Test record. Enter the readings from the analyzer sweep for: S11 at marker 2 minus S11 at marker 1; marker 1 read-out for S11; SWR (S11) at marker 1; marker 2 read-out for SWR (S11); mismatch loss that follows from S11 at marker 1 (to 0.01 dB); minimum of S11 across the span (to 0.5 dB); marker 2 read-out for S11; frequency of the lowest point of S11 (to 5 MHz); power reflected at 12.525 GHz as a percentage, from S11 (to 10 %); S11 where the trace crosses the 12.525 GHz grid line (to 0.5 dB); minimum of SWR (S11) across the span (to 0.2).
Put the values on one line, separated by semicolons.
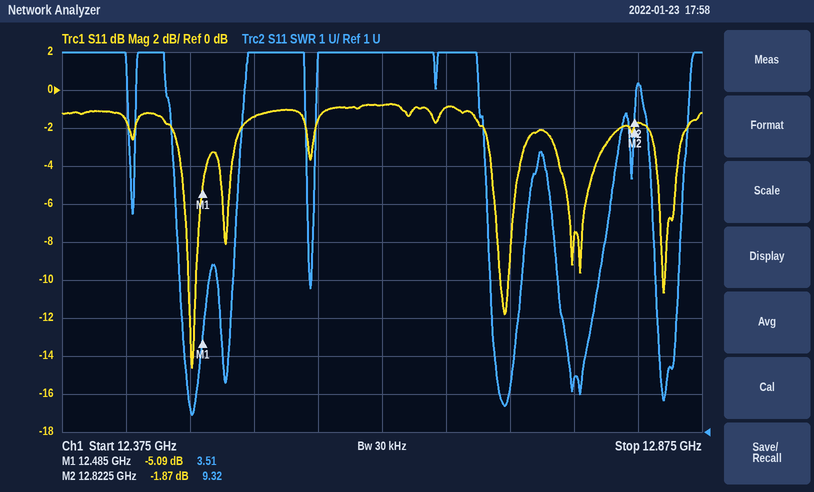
3.22 dB; -5.09 dB; 3.51; 9.32; 1.61 dB; -14.5 dB; -1.87 dB; 12.475 GHz; 70 %; -1.5 dB; 1.4
